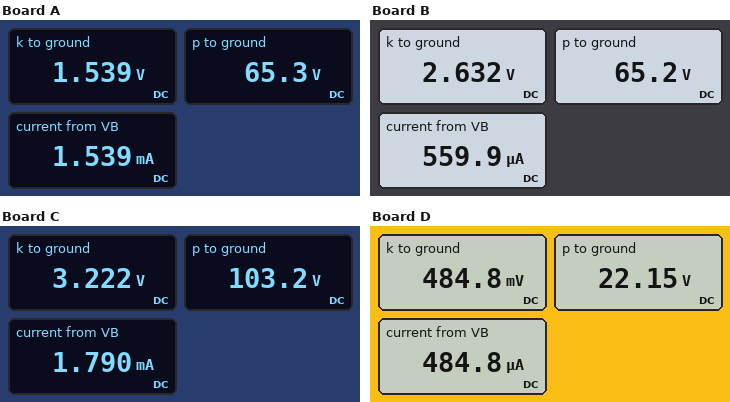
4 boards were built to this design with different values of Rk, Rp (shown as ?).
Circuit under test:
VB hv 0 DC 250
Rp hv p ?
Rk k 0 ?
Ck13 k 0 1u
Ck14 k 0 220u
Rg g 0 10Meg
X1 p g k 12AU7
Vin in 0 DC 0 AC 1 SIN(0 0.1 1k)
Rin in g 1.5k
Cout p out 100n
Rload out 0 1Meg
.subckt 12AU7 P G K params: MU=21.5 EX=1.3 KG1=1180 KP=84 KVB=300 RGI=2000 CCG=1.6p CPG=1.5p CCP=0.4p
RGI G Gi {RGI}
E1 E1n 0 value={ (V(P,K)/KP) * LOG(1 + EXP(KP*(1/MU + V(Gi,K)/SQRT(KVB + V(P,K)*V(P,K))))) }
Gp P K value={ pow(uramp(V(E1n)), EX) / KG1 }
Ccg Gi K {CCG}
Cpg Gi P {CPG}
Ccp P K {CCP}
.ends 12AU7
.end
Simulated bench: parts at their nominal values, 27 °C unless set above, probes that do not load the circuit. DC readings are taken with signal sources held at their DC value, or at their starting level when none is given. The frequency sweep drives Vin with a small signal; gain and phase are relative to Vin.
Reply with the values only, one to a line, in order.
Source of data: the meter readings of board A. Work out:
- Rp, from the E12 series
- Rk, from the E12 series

120 kΩ
1 kΩ
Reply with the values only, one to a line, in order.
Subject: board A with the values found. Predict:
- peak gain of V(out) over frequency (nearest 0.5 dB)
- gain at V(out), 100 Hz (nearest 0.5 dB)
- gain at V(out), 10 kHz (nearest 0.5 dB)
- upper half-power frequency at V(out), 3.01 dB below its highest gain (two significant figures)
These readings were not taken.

24.5 dB
24.5 dB
24.5 dB
1.3 MHz
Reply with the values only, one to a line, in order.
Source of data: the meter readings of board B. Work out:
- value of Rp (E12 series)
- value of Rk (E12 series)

330 kΩ
4.7 kΩ
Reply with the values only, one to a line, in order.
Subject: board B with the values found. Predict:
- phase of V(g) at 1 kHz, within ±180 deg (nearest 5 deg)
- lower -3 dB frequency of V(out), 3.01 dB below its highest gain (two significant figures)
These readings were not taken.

0 deg
1.6 Hz
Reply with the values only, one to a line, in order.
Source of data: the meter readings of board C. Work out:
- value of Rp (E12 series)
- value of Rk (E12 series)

82 kΩ
1.8 kΩ
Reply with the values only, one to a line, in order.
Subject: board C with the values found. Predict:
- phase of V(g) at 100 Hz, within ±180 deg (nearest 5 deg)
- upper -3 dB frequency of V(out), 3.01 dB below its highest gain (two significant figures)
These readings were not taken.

0 deg
1.4 MHz
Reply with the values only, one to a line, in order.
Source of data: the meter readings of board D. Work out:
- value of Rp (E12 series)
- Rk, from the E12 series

470 kΩ
1 kΩ
